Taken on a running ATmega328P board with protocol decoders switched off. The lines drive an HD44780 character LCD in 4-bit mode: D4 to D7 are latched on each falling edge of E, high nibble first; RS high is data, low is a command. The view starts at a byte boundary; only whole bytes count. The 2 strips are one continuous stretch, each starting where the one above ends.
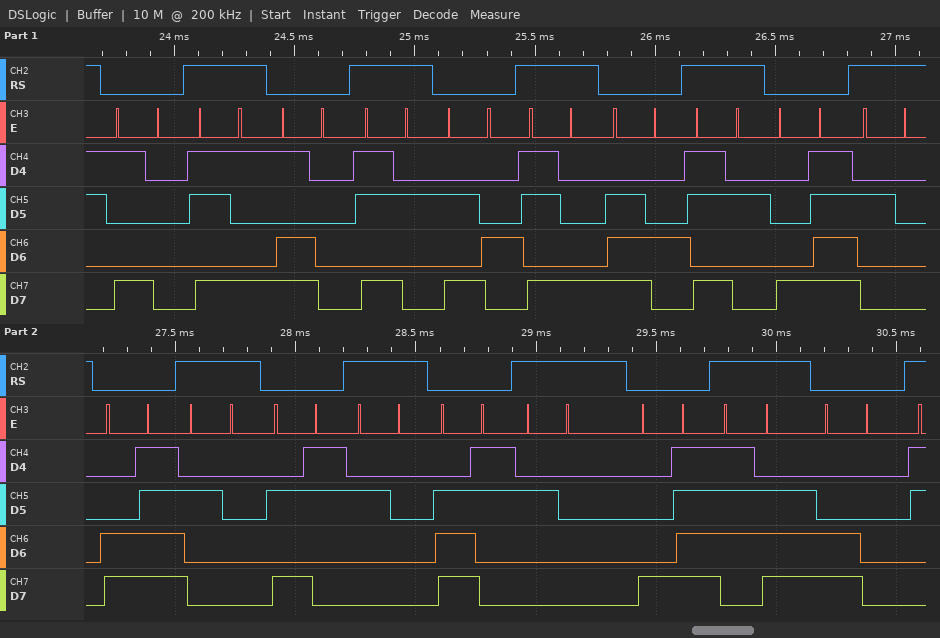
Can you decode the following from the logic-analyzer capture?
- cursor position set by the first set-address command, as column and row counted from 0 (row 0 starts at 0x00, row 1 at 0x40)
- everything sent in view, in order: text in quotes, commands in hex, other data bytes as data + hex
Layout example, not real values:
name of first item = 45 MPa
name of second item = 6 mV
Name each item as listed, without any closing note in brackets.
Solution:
cursor position set by the first set-address command, as column and row counted from 0 = column 16, row 0
everything sent in view, in order: text in quotes, commands in hex, other data bytes as data + hex = 0x90 data B9 0xD0 data B2 0xA4 data B8 0xE4 data B2 0x8F " " 0xCF " " 0xA3 " " 0xE3 " " 0x8F data 7E 0xC0
